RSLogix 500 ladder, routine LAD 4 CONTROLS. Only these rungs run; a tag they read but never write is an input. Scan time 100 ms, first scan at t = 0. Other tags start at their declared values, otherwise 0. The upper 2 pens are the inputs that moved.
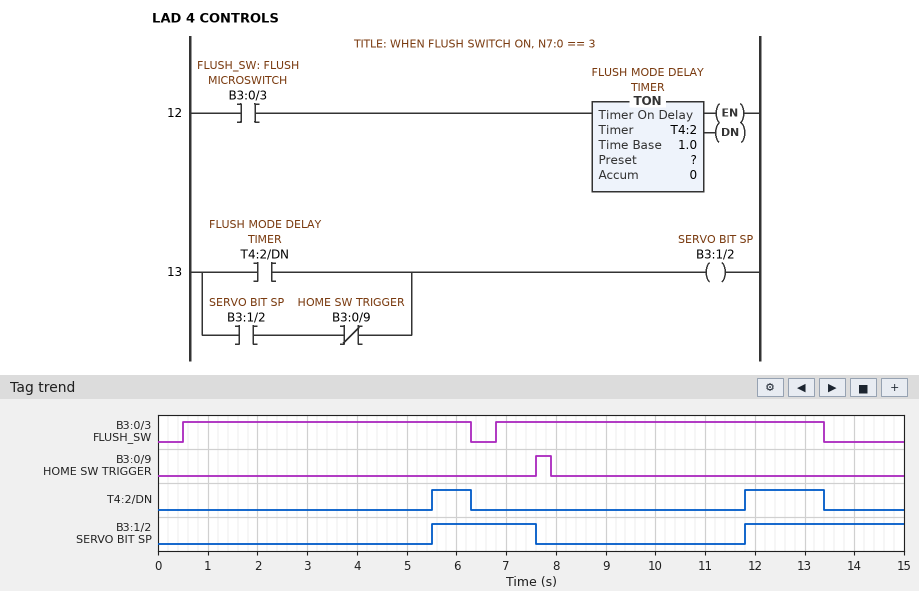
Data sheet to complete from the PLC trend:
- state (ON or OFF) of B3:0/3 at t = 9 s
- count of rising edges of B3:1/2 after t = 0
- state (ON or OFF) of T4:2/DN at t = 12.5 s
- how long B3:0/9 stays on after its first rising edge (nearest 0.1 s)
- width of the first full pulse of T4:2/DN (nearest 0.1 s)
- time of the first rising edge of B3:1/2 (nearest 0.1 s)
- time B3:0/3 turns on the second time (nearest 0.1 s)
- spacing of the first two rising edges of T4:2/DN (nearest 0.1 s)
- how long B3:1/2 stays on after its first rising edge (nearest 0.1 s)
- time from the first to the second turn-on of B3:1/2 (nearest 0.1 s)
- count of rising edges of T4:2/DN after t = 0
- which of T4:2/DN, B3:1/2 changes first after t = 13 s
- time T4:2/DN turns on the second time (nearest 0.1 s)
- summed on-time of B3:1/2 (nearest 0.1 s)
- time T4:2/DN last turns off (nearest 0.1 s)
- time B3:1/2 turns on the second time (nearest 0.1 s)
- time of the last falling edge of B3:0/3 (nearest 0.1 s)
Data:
ON
2
ON
0.3 s
0.8 s
5.5 s
6.8 s
6.3 s
2.1 s
6.3 s
2
T4:2/DN
11.8 s
5.3 s
13.4 s
11.8 s
13.4 s
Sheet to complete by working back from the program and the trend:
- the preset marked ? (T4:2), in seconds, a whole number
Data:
5 s
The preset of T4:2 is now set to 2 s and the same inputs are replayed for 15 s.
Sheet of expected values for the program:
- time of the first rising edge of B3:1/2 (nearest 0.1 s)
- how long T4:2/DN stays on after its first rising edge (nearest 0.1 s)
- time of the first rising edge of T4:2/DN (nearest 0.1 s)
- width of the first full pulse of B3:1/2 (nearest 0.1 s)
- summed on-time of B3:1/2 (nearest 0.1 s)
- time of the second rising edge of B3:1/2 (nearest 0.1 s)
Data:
2.5 s
3.8 s
2.5 s
5.1 s
11.3 s
8.8 s
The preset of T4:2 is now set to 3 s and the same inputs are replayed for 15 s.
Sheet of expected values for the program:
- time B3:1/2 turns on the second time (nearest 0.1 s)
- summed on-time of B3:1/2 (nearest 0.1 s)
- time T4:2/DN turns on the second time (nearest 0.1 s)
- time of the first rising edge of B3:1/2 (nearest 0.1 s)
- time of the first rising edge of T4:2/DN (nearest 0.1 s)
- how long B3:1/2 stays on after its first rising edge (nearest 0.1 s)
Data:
9.8 s
9.3 s
9.8 s
3.5 s
3.5 s
4.1 s
